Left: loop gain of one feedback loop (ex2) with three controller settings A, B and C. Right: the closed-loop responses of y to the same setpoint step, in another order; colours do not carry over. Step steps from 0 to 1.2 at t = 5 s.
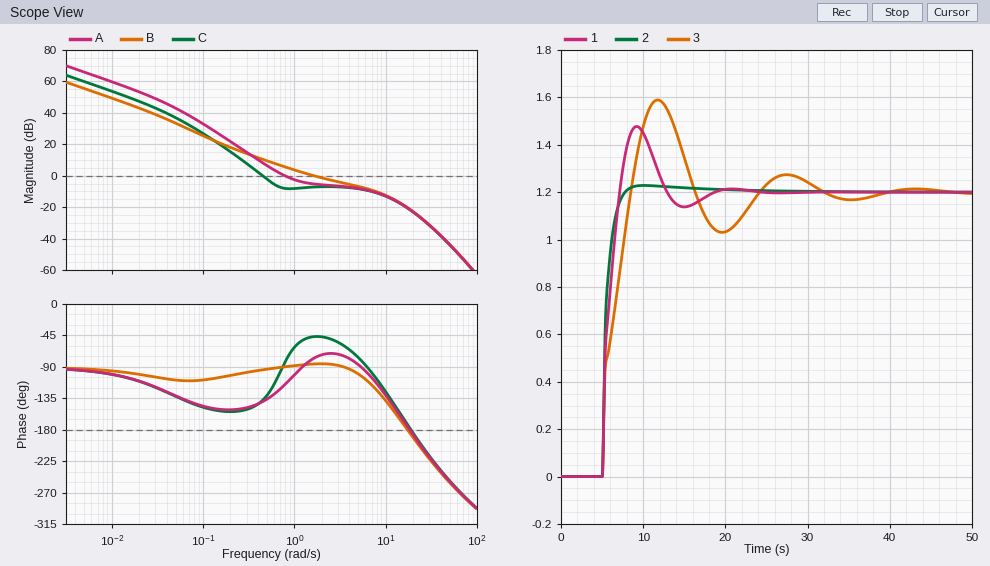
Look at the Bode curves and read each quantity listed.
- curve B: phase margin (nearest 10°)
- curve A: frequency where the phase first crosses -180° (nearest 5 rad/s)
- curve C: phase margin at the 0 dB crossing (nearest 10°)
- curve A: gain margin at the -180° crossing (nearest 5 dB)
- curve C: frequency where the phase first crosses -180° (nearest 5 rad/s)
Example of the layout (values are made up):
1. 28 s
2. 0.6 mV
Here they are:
1. 90°
2. 20 rad/s
3. 40°
4. 20 dB
5. 20 rad/s
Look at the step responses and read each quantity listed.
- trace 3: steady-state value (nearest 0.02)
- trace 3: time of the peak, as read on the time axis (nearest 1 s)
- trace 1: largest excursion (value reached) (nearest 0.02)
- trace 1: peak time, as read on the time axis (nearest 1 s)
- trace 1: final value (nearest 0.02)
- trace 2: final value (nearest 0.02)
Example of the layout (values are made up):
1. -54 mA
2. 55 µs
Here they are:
1. 1.20
2. 12 s
3. 1.48
4. 9 s
5. 1.20
6. 1.20
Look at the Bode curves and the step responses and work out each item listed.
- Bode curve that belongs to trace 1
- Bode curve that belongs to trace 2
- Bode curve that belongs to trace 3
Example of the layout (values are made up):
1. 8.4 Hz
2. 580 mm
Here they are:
1. A
2. B
3. C
